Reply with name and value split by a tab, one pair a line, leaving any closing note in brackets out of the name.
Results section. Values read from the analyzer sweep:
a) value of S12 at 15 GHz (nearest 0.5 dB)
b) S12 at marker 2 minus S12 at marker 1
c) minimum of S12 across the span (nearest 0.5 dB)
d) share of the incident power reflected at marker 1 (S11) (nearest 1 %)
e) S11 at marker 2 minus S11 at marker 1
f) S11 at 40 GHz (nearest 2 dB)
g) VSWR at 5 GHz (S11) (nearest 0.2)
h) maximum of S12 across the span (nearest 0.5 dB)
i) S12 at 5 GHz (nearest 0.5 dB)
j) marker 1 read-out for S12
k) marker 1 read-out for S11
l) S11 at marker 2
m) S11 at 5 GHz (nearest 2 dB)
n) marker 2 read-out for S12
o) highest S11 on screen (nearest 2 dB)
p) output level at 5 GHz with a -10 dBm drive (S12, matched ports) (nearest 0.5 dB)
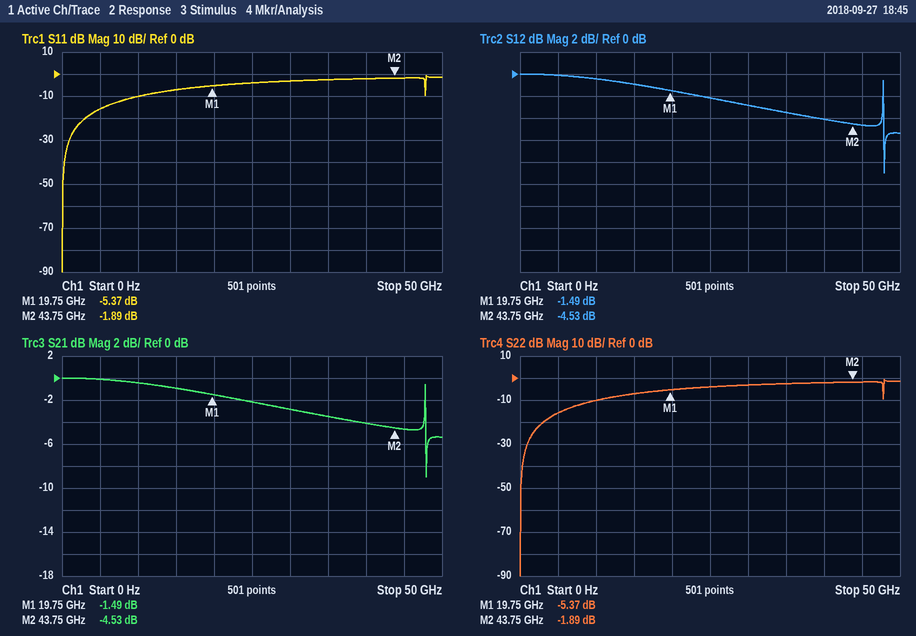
value of S12 at 15 GHz	-1.0 dB
S12 at marker 2 minus S12 at marker 1	-3.04 dB
minimum of S12 across the span	-9.0 dB
share of the incident power reflected at marker 1 (S11)	29 %
S11 at marker 2 minus S11 at marker 1	3.48 dB
S11 at 40 GHz	-2 dB
VSWR at 5 GHz (S11)	1.4
maximum of S12 across the span	0.0 dB
S12 at 5 GHz	0.0 dB
marker 1 read-out for S12	-1.49 dB
marker 1 read-out for S11	-5.37 dB
S11 at marker 2	-1.89 dB
S11 at 5 GHz	-16 dB
marker 2 read-out for S12	-4.53 dB
highest S11 on screen	0 dB
output level at 5 GHz with a -10 dBm drive (S12, matched ports)	-10.0 dBm
